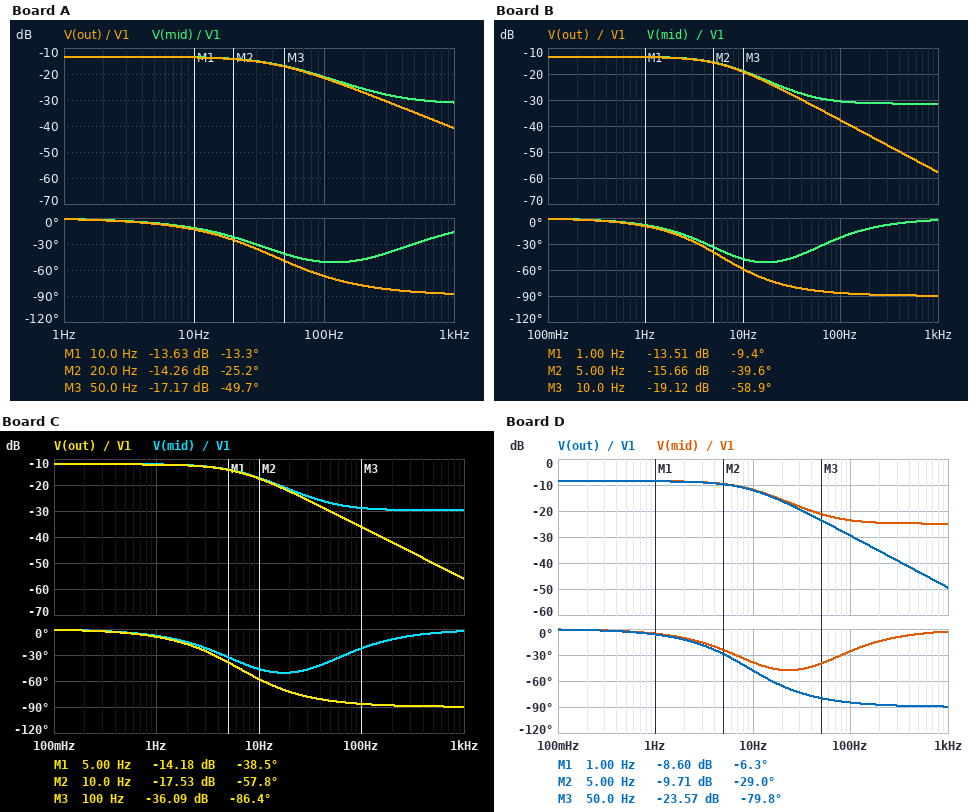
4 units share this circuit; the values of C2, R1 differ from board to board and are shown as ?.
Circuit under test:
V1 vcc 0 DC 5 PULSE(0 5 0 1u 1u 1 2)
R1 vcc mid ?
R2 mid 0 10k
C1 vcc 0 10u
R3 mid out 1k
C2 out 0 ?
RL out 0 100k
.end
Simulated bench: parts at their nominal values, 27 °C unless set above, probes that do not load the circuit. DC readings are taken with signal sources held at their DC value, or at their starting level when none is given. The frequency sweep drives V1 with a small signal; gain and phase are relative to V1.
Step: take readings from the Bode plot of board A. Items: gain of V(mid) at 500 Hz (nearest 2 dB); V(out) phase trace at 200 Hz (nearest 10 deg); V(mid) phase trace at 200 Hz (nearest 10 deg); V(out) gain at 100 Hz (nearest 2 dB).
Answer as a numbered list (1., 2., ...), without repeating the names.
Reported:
1. -30 dB
2. -80 deg
3. -50 deg
4. -22 dB
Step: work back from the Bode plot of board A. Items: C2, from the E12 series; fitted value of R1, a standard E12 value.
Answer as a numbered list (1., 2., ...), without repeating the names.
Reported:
1. 470 nF
2. 33 kΩ
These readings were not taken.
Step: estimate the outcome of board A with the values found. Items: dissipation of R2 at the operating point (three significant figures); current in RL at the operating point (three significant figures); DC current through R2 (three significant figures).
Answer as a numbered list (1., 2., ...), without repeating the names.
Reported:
1. 117 µW
2. 10.7 µA
3. 108 µA
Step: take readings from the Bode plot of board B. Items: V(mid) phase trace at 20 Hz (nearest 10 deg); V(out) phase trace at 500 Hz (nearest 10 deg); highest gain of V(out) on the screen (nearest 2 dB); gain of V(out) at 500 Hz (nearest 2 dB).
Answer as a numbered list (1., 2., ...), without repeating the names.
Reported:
1. -50 deg
2. -90 deg
3. -14 dB
4. -52 dB
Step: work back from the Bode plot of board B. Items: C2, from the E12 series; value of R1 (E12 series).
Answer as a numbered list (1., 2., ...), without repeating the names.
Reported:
1. 3.3 µF
2. 33 kΩ
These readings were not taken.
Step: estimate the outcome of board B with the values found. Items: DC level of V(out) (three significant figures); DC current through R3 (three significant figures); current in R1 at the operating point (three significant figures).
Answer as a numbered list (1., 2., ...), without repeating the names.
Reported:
1. 1.07 V
2. 10.7 µA
3. 119 µA
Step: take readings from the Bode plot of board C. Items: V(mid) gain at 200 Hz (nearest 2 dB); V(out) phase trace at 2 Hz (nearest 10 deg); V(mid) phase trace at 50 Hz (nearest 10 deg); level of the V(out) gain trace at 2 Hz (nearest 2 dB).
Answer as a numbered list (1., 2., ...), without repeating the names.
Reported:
1. -30 dB
2. -20 deg
3. -40 deg
4. -12 dB
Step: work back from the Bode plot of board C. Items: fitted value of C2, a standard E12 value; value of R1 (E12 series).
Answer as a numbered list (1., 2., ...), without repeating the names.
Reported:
1. 3.3 µF
2. 27 kΩ
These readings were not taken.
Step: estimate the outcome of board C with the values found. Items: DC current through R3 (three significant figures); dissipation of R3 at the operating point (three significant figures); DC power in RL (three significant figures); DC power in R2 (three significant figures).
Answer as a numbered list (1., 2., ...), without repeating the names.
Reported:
1. 12.5 µA
2. 156 nW
3. 15.6 µW
4. 159 µW
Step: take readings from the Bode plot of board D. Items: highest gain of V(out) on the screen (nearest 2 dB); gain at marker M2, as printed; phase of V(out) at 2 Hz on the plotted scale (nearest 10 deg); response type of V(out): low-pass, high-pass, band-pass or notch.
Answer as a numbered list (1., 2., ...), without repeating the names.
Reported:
1. -8 dB
2. -9.71 dB
3. -10 deg
4. low-pass
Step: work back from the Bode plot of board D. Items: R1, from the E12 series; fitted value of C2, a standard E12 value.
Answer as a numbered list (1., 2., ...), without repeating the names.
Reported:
1. 15 kΩ
2. 2.7 µF
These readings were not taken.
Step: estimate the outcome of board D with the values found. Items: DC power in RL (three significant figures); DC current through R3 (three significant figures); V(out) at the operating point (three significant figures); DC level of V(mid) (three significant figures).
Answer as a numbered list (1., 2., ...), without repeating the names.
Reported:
1. 34.9 µW
2. 18.7 µA
3. 1.87 V
4. 1.89 V
